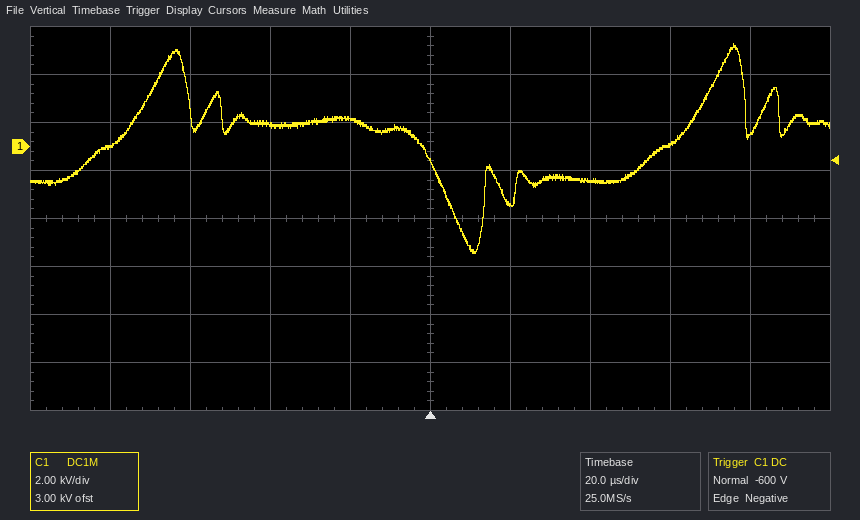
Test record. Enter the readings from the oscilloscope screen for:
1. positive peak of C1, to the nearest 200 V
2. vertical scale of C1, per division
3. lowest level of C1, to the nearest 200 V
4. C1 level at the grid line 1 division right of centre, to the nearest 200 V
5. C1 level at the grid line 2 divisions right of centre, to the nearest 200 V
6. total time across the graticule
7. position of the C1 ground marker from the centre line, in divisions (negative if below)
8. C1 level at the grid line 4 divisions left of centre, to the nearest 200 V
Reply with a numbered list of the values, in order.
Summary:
1. 4.2 kV
2. 2 kV
3. -4.4 kV
4. -2.4 kV
5. -1.4 kV
6. 200 µs
7. +1.5 div
8. 0.0 kV
